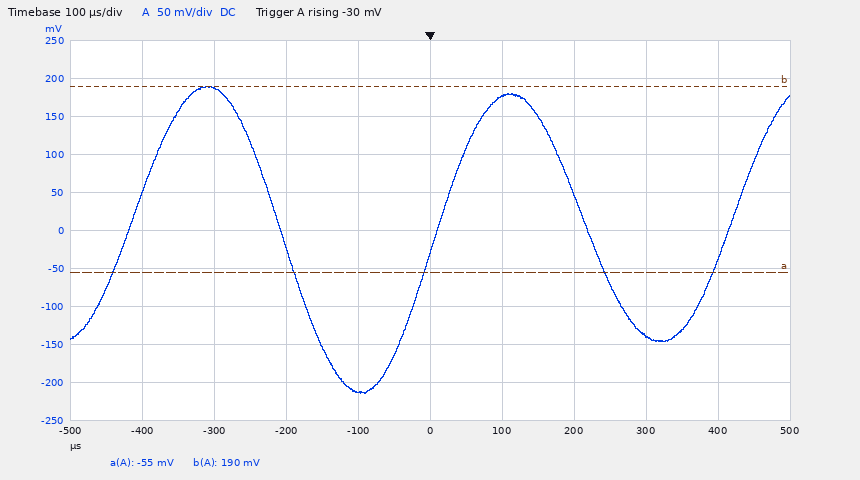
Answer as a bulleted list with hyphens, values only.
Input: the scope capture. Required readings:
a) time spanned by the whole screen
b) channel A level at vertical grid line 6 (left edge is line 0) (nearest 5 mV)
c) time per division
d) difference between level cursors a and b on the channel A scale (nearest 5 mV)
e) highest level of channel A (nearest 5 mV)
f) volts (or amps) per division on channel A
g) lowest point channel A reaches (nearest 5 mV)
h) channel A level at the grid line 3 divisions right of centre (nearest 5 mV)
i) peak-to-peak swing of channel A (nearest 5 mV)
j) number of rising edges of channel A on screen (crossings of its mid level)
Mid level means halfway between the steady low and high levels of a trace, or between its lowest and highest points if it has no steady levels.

- 1 ms
- 175 mV
- 100 µs
- 245 mV
- 190 mV
- 50 mV
- -215 mV
- -140 mV
- 405 mV
- 3
